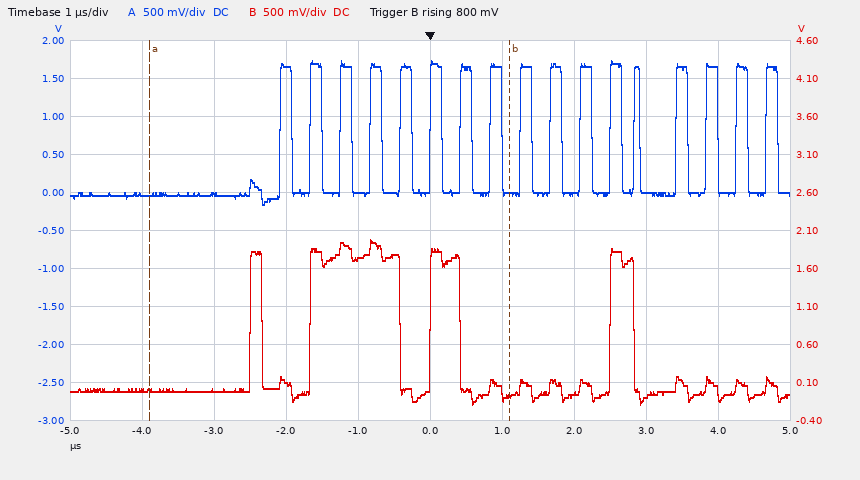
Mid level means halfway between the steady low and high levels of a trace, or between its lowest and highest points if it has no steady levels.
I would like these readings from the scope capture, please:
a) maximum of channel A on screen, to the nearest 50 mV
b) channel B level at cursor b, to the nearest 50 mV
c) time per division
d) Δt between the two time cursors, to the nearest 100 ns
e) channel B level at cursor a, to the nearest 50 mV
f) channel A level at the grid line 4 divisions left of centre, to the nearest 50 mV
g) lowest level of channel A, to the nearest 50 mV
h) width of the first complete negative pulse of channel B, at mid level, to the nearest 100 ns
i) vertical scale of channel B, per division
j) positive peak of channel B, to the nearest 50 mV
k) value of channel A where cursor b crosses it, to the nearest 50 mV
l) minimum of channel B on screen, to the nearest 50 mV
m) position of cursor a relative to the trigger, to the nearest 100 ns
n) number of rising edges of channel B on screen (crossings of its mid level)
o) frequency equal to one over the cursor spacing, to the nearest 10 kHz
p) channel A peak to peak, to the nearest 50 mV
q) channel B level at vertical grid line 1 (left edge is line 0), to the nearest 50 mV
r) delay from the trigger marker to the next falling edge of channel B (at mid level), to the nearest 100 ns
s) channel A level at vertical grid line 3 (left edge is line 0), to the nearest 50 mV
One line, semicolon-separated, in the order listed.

1.75 V; -100 mV; 1 µs; 5.0 µs; 0 mV; 0 mV; -150 mV; 700 ns; 500 mV; 2.00 V; 0 mV; -200 mV; -3.9 µs; 4; 200 kHz; 1.90 V; 0 mV; 400 ns; 1.65 V
